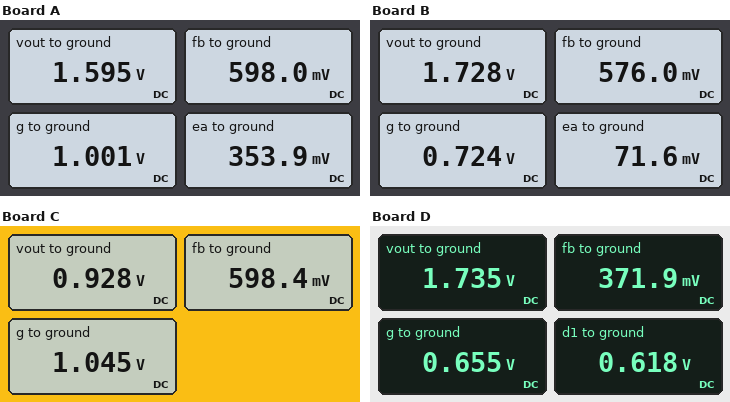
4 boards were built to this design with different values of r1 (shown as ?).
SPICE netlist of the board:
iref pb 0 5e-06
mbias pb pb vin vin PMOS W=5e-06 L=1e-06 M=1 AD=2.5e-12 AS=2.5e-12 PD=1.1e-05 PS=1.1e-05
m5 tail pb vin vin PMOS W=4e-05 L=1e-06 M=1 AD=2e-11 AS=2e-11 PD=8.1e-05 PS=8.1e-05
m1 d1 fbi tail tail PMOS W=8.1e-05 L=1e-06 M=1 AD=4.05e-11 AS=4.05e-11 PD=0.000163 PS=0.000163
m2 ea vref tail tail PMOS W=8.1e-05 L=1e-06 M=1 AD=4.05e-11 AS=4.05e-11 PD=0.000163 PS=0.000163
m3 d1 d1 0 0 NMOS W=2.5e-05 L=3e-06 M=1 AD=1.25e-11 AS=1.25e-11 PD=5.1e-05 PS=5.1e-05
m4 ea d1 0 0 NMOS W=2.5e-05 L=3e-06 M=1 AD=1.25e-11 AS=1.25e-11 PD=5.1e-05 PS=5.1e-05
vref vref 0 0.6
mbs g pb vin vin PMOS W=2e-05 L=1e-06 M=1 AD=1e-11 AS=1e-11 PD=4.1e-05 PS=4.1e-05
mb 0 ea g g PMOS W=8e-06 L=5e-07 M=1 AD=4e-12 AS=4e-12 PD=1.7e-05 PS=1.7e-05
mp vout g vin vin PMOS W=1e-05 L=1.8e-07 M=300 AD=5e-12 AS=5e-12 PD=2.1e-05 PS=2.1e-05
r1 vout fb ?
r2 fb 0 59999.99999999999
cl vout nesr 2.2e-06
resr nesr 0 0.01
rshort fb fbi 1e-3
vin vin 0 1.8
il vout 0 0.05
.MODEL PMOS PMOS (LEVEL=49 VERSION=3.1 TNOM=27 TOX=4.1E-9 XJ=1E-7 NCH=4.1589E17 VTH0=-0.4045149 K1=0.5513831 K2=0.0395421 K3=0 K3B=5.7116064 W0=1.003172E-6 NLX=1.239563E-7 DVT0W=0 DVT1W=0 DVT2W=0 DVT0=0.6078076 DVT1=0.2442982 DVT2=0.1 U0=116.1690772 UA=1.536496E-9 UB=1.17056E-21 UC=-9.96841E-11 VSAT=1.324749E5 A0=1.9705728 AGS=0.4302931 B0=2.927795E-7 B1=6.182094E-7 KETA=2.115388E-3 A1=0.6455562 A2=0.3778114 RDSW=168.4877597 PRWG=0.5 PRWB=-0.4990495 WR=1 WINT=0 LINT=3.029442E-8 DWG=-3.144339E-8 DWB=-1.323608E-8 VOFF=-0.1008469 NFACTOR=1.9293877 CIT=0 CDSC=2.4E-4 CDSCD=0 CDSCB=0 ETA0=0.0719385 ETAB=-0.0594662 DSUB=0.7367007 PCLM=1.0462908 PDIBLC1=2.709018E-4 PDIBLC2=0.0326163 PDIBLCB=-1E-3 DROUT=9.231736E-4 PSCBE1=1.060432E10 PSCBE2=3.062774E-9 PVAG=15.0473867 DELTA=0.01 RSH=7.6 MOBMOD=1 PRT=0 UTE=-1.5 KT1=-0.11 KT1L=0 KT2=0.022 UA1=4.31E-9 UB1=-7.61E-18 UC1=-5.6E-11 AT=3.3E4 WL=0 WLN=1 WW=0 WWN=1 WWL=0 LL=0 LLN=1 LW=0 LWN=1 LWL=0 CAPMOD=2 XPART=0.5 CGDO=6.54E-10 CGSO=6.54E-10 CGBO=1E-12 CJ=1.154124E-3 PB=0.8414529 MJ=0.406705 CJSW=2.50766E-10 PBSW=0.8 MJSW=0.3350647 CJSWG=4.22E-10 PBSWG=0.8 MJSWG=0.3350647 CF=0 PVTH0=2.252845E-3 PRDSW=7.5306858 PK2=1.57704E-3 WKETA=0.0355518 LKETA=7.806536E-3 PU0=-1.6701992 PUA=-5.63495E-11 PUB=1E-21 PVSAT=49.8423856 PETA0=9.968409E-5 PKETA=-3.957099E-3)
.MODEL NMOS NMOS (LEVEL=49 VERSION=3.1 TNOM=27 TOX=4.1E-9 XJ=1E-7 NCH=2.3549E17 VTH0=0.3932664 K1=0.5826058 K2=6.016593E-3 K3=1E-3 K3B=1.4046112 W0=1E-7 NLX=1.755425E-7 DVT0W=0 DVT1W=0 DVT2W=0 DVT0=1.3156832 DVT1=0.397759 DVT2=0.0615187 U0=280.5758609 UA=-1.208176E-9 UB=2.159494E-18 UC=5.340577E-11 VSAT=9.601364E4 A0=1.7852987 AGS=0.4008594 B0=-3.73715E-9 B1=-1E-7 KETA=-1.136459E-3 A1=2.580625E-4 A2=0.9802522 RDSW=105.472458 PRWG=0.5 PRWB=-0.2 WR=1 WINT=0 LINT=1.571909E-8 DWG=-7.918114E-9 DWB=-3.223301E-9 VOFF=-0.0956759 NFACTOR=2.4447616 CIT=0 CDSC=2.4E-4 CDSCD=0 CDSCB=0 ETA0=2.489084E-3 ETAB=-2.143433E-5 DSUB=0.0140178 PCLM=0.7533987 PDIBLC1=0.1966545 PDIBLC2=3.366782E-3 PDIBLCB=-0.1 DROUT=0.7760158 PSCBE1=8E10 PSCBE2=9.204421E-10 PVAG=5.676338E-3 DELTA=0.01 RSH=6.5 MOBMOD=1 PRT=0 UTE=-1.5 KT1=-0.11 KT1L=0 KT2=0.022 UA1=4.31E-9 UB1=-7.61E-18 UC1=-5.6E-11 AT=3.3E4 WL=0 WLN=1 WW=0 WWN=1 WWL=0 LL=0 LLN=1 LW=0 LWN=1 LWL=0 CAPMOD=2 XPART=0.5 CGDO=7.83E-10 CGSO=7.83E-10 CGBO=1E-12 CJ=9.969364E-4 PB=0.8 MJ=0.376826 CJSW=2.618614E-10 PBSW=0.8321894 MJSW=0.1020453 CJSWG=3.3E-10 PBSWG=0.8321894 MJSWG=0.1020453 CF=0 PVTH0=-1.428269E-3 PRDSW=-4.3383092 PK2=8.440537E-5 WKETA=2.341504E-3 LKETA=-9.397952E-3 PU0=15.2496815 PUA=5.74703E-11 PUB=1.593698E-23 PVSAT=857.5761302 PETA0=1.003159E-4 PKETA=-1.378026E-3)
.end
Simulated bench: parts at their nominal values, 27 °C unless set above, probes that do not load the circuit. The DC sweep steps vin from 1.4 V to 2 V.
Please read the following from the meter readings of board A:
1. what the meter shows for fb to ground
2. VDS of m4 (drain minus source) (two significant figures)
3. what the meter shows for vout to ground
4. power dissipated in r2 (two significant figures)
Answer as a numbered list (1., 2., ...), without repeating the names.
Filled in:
1. 598.0 mV
2. 350 mV
3. 1.595 V
4. 6.0 µW
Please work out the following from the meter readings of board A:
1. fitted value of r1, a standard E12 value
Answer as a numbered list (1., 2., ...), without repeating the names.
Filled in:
1. 100 kΩ
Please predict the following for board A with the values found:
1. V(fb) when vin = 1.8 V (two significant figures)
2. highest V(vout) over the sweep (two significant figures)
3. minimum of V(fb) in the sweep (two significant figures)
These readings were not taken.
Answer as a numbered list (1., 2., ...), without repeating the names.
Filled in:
1. 600 mV
2. 1.6 V
3. 130 mV
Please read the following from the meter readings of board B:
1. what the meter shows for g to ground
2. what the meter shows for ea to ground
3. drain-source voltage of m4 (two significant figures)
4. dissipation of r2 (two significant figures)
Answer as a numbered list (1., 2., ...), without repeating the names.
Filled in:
1. 0.724 V
2. 71.6 mV
3. 72 mV
4. 5.5 µW
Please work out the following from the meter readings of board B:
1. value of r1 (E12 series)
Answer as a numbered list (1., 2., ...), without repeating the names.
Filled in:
1. 120 kΩ
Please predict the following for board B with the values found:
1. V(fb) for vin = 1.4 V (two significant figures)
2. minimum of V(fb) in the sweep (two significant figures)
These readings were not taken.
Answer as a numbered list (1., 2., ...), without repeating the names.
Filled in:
1. 120 mV
2. 120 mV
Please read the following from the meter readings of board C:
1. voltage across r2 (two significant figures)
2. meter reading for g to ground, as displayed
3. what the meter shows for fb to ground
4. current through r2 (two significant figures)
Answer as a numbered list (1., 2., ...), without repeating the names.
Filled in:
1. 600 mV
2. 1.045 V
3. 598.4 mV
4. 10 µA
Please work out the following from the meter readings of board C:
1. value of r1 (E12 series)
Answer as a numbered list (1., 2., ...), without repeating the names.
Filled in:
1. 33 kΩ
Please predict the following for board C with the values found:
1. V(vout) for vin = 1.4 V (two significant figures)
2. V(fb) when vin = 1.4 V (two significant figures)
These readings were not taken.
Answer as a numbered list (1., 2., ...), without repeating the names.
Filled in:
1. 350 mV
2. 230 mV
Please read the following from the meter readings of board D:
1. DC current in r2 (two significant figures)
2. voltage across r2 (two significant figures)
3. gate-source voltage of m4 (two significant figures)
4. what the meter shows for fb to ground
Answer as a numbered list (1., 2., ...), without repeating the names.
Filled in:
1. 6.2 µA
2. 370 mV
3. 620 mV
4. 371.9 mV
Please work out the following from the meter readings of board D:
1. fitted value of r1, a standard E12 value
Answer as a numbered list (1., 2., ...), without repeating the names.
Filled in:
1. 220 kΩ
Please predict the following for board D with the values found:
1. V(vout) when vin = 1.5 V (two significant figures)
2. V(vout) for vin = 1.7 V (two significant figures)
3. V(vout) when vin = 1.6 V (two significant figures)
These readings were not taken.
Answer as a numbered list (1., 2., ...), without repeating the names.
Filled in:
1. 1.4 V
2. 1.6 V
3. 1.5 V
